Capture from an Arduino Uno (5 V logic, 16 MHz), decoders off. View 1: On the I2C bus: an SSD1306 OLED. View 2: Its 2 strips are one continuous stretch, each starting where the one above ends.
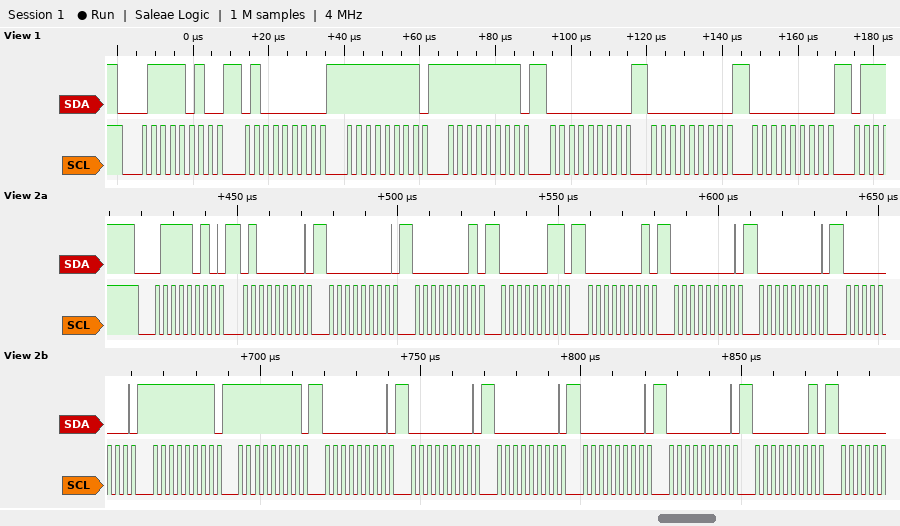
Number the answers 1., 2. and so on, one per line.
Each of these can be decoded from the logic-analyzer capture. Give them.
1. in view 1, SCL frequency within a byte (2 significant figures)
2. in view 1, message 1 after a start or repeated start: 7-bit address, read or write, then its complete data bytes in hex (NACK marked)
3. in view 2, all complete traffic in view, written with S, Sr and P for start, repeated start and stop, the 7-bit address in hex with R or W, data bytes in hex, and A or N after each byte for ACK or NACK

1. 400 kHz
2. 0x3D write: 40 FF FF 00 00 00
3. S 3DW A 40 A 00 A 01 A 03 A 01 A 00 A 00 A 00 A FF A FF A 00 A 00 A 00 A 00 A 00 A 01 A
